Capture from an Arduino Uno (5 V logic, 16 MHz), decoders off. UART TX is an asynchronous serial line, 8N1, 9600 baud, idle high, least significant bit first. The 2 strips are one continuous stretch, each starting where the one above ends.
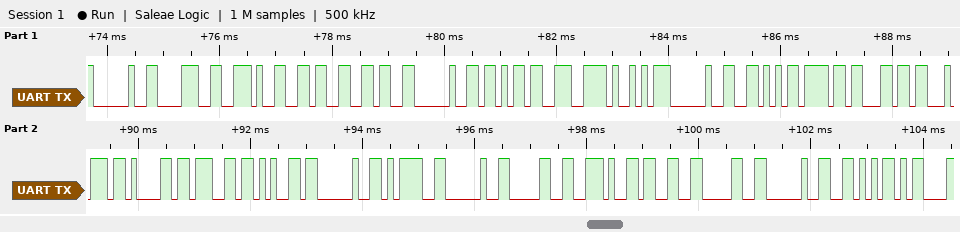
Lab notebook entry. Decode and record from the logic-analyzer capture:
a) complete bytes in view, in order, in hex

0x20 0x38 0x2E 0x36 0x36 0x20 0x6B 0xCE 0xA9 0x20 0x56 0x6F 0x6C 0x74 0x61 0x67 0x65 0x20 0x3D 0x20 0x30 0x2E 0x33 0x30 0x20 0x56 0x0D
